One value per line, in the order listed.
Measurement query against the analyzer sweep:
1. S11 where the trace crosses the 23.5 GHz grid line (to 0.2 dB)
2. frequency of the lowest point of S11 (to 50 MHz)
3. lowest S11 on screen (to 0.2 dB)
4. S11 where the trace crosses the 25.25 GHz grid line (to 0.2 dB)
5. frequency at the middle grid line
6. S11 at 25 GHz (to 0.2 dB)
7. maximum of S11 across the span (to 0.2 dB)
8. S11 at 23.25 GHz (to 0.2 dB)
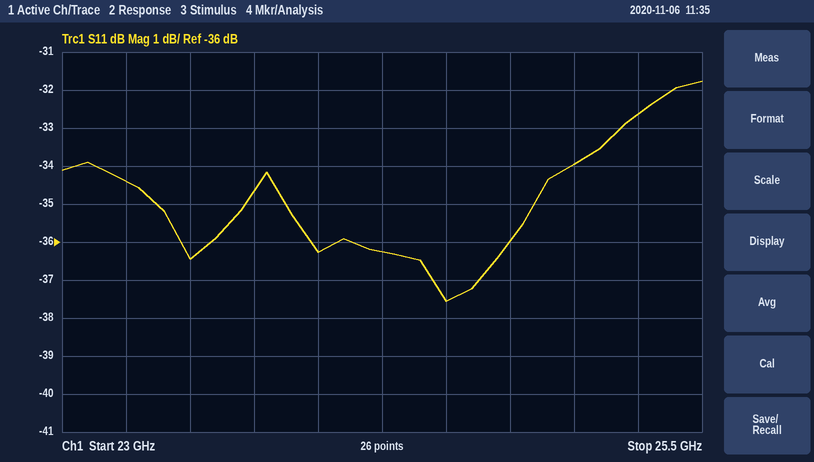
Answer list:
-36.4 dB
24.50 GHz
-37.6 dB
-32.6 dB
24.25 GHz
-34.0 dB
-31.8 dB
-34.4 dB
